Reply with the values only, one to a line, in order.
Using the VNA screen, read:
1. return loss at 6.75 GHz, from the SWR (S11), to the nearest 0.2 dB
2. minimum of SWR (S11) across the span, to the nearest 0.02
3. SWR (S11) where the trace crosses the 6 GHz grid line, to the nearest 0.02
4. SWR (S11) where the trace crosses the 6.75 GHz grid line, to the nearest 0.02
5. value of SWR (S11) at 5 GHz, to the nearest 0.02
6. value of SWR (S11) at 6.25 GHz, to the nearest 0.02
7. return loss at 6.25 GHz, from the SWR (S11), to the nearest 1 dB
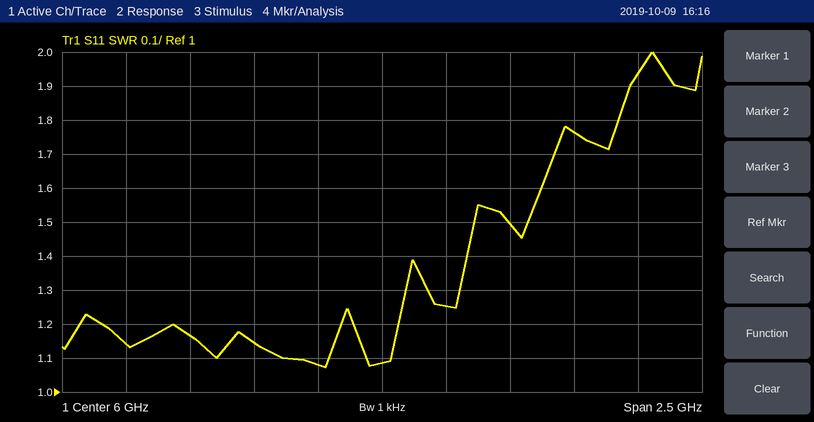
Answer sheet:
11.2 dB
1.08
1.08
1.76
1.14
1.26
19 dB
